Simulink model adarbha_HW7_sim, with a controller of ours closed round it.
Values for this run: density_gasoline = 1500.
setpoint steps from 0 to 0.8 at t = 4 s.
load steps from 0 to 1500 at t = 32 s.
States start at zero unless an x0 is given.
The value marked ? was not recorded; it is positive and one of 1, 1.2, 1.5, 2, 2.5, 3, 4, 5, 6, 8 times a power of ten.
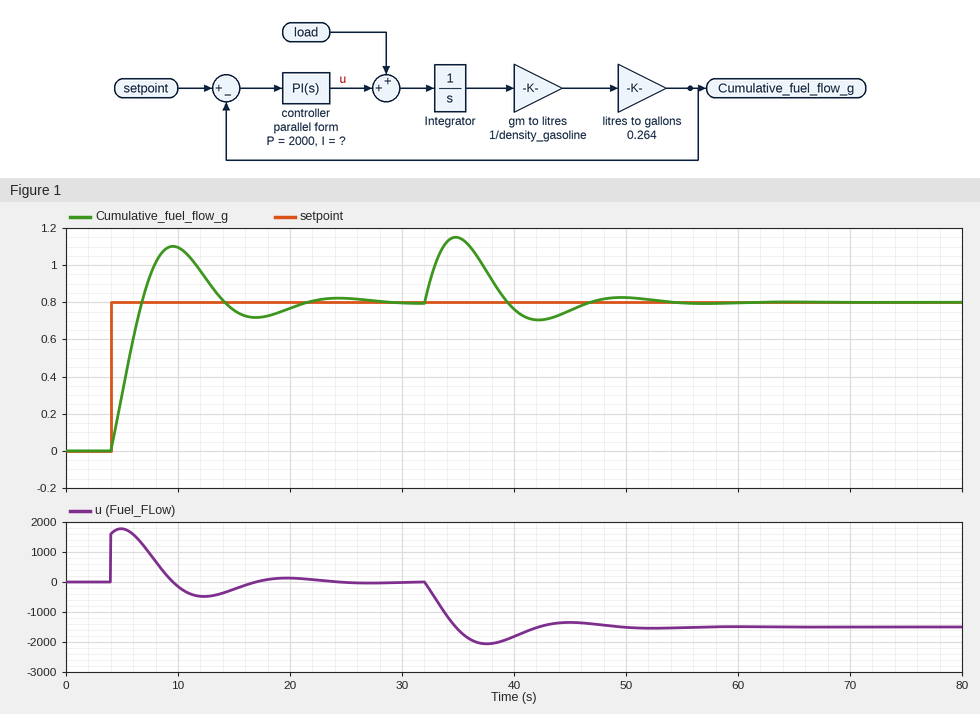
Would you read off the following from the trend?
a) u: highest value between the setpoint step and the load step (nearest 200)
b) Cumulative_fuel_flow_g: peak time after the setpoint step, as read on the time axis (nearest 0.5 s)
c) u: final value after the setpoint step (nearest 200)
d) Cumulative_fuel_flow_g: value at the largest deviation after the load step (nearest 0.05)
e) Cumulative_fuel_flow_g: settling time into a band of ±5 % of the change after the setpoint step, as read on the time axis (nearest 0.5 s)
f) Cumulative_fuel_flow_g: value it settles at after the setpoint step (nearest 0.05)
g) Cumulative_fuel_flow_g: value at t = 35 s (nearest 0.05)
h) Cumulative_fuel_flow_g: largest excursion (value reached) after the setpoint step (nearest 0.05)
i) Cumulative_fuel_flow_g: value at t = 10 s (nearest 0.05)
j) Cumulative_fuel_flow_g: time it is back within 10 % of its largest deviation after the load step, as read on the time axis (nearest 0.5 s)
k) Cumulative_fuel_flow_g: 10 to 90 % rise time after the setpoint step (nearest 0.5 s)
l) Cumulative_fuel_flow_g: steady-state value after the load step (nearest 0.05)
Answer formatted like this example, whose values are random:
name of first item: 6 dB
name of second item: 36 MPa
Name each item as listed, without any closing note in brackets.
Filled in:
u: highest value between the setpoint step and the load step: 1800
Cumulative_fuel_flow_g: peak time after the setpoint step, as read on the time axis: 9.5 s
u: final value after the setpoint step: 0
Cumulative_fuel_flow_g: value at the largest deviation after the load step: 1.15
Cumulative_fuel_flow_g: settling time into a band of ±5 % of the change after the setpoint step, as read on the time axis: 19.5 s
Cumulative_fuel_flow_g: value it settles at after the setpoint step: 0.80
Cumulative_fuel_flow_g: value at t = 35 s: 1.15
Cumulative_fuel_flow_g: largest excursion (value reached) after the setpoint step: 1.10
Cumulative_fuel_flow_g: value at t = 10 s: 1.10
Cumulative_fuel_flow_g: time it is back within 10 % of its largest deviation after the load step, as read on the time axis: 45.5 s
Cumulative_fuel_flow_g: 10 to 90 % rise time after the setpoint step: 2.0 s
Cumulative_fuel_flow_g: steady-state value after the load step: 0.80
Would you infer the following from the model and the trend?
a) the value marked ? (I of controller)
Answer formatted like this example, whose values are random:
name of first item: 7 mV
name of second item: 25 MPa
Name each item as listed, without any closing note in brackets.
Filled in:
the value marked ?: 1200
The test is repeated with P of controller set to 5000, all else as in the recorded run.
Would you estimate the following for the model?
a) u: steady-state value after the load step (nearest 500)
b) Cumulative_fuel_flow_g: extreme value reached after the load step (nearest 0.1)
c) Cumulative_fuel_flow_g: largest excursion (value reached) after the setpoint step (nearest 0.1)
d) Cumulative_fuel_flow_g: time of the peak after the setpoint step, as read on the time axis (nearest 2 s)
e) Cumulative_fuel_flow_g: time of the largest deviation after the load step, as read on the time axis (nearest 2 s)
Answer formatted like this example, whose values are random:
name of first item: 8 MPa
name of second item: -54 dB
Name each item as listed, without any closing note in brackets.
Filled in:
u: steady-state value after the load step: -1500
Cumulative_fuel_flow_g: extreme value reached after the load step: 1.0
Cumulative_fuel_flow_g: largest excursion (value reached) after the setpoint step: 0.9
Cumulative_fuel_flow_g: time of the peak after the setpoint step, as read on the time axis: 8 s
Cumulative_fuel_flow_g: time of the largest deviation after the load step, as read on the time axis: 34 s
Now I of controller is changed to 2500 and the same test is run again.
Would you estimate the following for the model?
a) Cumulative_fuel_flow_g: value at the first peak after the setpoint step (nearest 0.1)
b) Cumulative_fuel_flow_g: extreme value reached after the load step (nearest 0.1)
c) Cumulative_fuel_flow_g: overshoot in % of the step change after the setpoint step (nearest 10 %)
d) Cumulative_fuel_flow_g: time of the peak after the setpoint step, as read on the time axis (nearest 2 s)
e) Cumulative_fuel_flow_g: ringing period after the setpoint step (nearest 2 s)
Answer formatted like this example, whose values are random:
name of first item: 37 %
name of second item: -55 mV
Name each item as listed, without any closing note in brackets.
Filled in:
Cumulative_fuel_flow_g: value at the first peak after the setpoint step: 1.2
Cumulative_fuel_flow_g: extreme value reached after the load step: 1.1
Cumulative_fuel_flow_g: overshoot in % of the step change after the setpoint step: 50 %
Cumulative_fuel_flow_g: time of the peak after the setpoint step, as read on the time axis: 8 s
Cumulative_fuel_flow_g: ringing period after the setpoint step: 10 s
